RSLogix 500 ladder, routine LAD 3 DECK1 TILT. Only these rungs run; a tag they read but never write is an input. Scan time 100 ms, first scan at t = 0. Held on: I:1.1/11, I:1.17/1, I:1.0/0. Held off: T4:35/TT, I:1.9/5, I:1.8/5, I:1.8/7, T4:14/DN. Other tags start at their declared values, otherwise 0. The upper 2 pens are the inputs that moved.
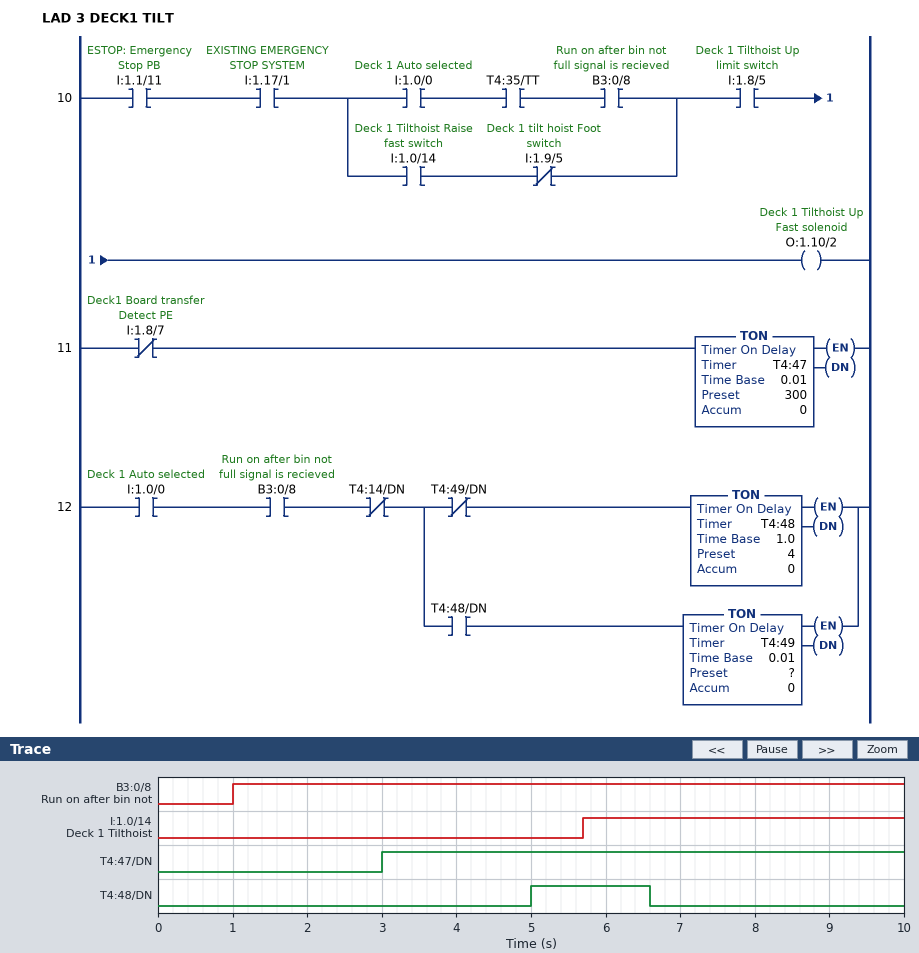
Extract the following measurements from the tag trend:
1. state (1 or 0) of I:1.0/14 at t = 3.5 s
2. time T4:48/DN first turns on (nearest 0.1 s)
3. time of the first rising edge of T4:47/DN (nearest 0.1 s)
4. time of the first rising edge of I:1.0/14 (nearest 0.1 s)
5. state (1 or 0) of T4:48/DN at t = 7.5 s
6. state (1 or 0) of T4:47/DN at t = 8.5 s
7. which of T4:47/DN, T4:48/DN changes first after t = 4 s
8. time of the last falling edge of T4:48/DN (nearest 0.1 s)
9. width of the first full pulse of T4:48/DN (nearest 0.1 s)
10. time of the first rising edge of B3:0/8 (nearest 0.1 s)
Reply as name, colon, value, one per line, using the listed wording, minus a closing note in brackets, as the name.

state (1 or 0) of I:1.0/14 at t = 3.5 s: 0
time T4:48/DN first turns on: 5.0 s
time of the first rising edge of T4:47/DN: 3.0 s
time of the first rising edge of I:1.0/14: 5.7 s
state (1 or 0) of T4:48/DN at t = 7.5 s: 0
state (1 or 0) of T4:47/DN at t = 8.5 s: 1
which of T4:47/DN, T4:48/DN changes first after t = 4 s: T4:48/DN
time of the last falling edge of T4:48/DN: 6.6 s
width of the first full pulse of T4:48/DN: 1.6 s
time of the first rising edge of B3:0/8: 1.0 s
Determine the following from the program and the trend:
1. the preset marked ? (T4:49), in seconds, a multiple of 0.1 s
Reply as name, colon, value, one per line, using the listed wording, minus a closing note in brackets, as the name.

the preset marked ? (T4:49), in seconds, a multiple of 0.1 s: 1.5 s
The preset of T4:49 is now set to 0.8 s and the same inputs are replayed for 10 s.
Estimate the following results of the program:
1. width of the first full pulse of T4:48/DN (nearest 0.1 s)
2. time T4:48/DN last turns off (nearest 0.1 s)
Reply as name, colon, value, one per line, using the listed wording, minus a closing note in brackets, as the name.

width of the first full pulse of T4:48/DN: 0.9 s
time T4:48/DN last turns off: 5.9 s
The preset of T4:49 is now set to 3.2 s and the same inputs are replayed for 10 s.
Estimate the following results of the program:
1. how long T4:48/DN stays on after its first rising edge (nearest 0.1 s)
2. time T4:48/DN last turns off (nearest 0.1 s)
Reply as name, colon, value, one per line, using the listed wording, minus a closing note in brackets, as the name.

how long T4:48/DN stays on after its first rising edge: 3.3 s
time T4:48/DN last turns off: 8.3 s
